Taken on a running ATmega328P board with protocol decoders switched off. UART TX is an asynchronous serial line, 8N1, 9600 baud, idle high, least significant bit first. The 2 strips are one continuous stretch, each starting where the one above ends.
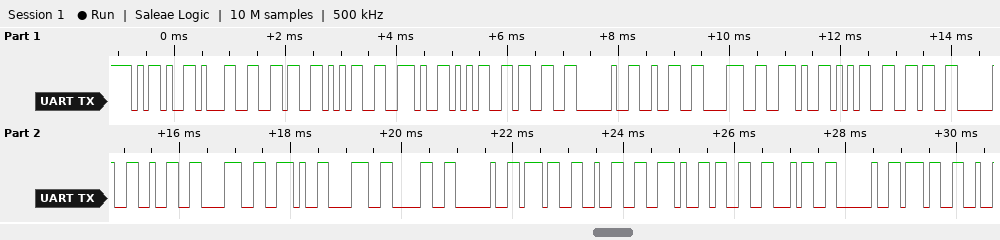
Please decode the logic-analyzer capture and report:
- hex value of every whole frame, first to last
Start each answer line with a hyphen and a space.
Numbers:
- 2D 31 36 35 2E 35 33 20 32 38 2E 35 36 20 32 38 2E 38 30 20 37 32 2E 33 34 20 37
